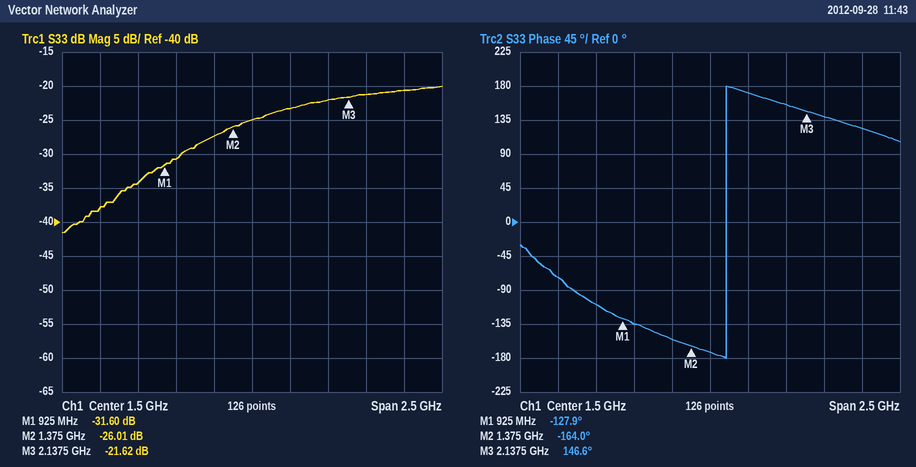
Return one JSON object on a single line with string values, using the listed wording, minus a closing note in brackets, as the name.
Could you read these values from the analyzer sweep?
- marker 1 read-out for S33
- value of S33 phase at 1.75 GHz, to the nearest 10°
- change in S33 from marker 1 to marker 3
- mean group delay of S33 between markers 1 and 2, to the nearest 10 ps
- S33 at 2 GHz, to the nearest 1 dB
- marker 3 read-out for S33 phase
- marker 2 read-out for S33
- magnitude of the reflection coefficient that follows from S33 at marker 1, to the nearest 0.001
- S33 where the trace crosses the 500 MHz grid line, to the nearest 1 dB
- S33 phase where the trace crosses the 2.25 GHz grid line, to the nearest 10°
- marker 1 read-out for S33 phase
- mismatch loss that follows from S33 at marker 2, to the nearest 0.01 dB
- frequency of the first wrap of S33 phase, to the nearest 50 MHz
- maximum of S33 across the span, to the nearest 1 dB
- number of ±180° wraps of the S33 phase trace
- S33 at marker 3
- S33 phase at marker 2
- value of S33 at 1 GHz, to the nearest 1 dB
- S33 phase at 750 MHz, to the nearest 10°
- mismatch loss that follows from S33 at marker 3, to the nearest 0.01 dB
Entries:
{"marker 1 read-out for S33": "-31.60 dB", "value of S33 phase at 1.75 GHz, to the nearest 10°": "170°", "change in S33 from marker 1 to marker 3": "9.98 dB", "mean group delay of S33 between markers 1 and 2, to the nearest 10 ps": "220 ps", "S33 at 2 GHz, to the nearest 1 dB": "-22 dB", "marker 3 read-out for S33 phase": "146.6°", "marker 2 read-out for S33": "-26.01 dB", "magnitude of the reflection coefficient that follows from S33 at marker 1, to the nearest 0.001": "0.026", "S33 where the trace crosses the 500 MHz grid line, to the nearest 1 dB": "-38 dB", "S33 phase where the trace crosses the 2.25 GHz grid line, to the nearest 10°": "140°", "marker 1 read-out for S33 phase": "-127.9°", "mismatch loss that follows from S33 at marker 2, to the nearest 0.01 dB": "0.01 dB", "frequency of the first wrap of S33 phase, to the nearest 50 MHz": "1.60 GHz", "maximum of S33 across the span, to the nearest 1 dB": "-20 dB", "number of ±180° wraps of the S33 phase trace": "1", "S33 at marker 3": "-21.62 dB", "S33 phase at marker 2": "-164.0°", "value of S33 at 1 GHz, to the nearest 1 dB": "-31 dB", "S33 phase at 750 MHz, to the nearest 10°": "-110°", "mismatch loss that follows from S33 at marker 3, to the nearest 0.01 dB": "0.03 dB"}
